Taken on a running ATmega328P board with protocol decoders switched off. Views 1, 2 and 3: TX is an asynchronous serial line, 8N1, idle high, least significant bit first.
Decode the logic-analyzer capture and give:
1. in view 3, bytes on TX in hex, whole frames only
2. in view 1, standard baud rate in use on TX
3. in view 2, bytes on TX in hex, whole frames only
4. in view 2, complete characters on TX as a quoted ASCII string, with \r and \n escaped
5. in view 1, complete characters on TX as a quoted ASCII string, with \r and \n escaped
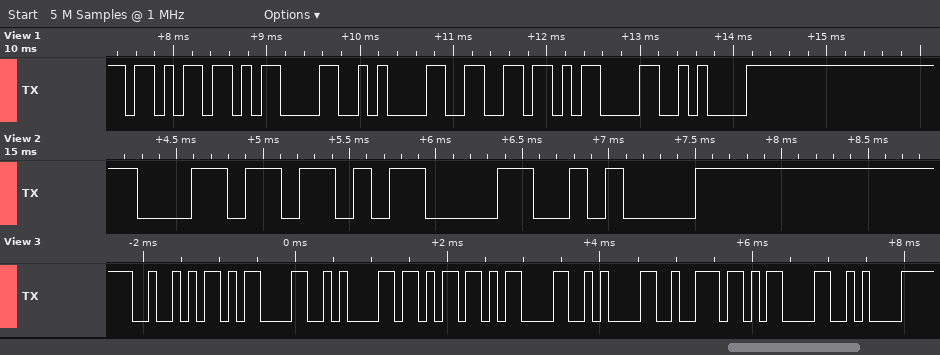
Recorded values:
0x52 0x0D 0x0A 0x6B 0x0D 0x0A 0x72 0x0D 0x0A
9600 baud
6C 0D 0A
"l\r\n"
"k\r\nf\r\n"
